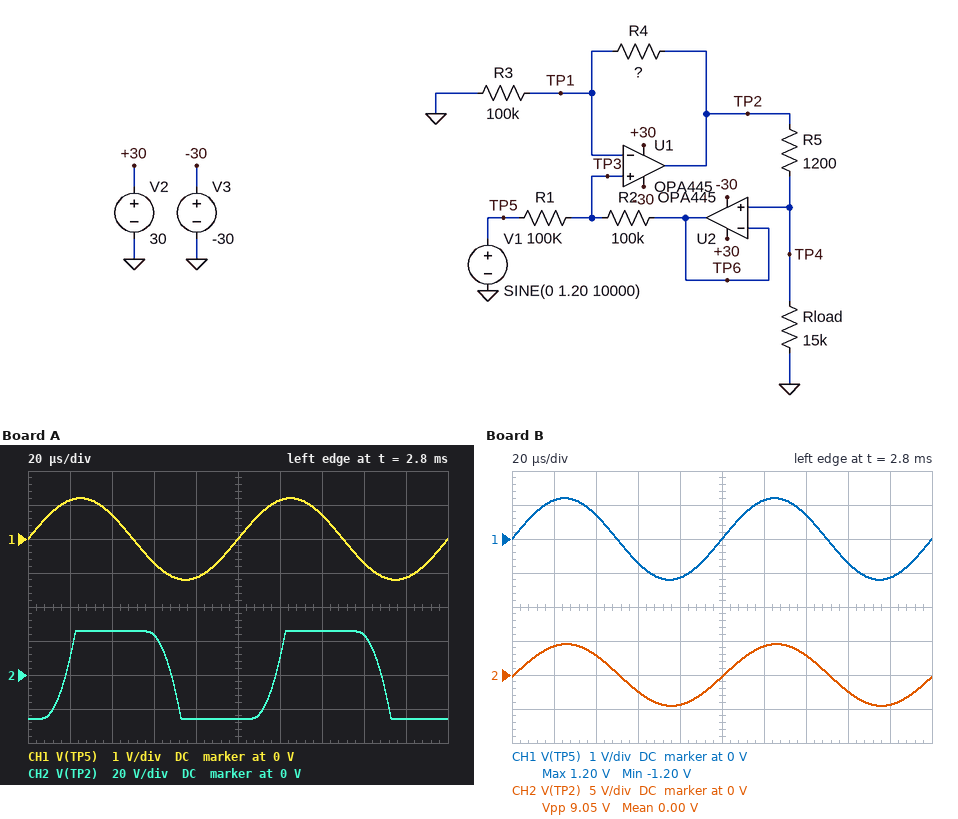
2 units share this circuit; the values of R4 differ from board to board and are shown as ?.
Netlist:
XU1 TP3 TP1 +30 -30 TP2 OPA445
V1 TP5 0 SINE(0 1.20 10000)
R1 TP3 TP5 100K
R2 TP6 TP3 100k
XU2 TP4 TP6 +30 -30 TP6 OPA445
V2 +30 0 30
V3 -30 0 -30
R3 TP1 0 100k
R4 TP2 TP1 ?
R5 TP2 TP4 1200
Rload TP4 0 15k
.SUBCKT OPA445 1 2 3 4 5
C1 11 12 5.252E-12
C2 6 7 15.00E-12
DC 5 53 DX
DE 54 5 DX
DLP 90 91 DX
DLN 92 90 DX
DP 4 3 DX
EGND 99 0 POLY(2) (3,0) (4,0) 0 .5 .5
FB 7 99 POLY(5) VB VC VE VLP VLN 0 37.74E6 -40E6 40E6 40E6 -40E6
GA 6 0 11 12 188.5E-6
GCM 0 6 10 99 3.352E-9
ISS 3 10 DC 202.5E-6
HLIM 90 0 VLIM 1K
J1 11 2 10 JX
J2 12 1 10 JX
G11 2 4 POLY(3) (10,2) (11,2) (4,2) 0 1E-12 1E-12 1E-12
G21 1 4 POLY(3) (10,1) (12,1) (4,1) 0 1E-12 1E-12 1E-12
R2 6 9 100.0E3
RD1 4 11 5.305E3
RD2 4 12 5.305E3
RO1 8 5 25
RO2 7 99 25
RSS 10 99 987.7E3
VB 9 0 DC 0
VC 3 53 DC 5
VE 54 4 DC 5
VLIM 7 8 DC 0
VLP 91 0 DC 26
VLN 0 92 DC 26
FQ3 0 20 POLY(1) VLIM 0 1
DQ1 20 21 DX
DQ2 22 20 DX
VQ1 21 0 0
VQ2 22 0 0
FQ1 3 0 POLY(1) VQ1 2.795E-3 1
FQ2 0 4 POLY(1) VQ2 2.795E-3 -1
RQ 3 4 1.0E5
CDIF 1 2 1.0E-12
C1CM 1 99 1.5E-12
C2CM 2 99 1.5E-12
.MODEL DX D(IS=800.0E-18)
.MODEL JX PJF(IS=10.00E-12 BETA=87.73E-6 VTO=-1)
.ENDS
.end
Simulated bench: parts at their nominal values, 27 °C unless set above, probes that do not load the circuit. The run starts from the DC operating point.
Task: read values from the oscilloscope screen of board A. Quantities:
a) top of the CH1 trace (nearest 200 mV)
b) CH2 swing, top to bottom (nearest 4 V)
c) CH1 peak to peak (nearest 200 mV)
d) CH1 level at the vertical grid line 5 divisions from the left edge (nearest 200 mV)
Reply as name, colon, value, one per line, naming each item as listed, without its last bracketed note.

top of the CH1 trace: 1.2 V
CH2 swing, top to bottom: 52 V
CH1 peak to peak: 2.4 V
CH1 level at the vertical grid line 5 divisions from the left edge: 0 V
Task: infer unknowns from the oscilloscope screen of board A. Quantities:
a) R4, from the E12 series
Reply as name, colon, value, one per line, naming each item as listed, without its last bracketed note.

R4, from the E12 series: 120 kΩ
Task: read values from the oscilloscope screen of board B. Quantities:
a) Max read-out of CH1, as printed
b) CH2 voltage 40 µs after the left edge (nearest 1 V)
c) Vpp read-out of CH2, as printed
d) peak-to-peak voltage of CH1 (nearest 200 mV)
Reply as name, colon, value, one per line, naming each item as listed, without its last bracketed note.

Max read-out of CH1, as printed: 1.20 V
CH2 voltage 40 µs after the left edge: 3 V
Vpp read-out of CH2, as printed: 9.05 V
peak-to-peak voltage of CH1: 2.4 V
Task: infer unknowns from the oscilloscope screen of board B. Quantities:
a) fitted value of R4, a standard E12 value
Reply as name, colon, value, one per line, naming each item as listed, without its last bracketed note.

fitted value of R4, a standard E12 value: 68 kΩ
